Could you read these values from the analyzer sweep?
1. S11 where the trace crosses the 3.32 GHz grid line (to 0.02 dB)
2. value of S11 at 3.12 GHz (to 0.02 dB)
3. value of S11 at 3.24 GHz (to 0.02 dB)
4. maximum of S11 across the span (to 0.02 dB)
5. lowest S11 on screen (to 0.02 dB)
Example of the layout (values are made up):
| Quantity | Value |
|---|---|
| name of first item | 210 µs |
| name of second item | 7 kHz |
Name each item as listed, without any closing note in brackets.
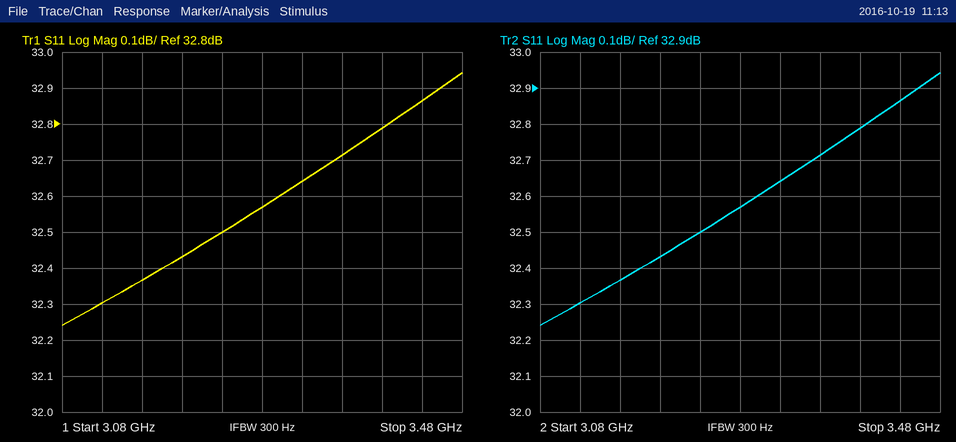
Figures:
| Quantity | Value |
|---|---|
| S11 where the trace crosses the 3.32 GHz grid line | 32.64 dB |
| value of S11 at 3.12 GHz | 32.30 dB |
| value of S11 at 3.24 GHz | 32.50 dB |
| maximum of S11 across the span | 32.94 dB |
| lowest S11 on screen | 32.24 dB |
